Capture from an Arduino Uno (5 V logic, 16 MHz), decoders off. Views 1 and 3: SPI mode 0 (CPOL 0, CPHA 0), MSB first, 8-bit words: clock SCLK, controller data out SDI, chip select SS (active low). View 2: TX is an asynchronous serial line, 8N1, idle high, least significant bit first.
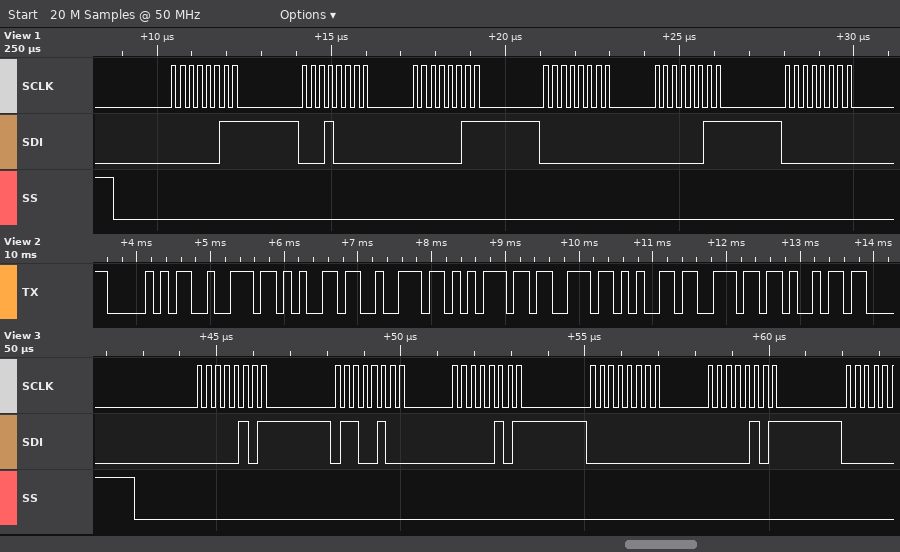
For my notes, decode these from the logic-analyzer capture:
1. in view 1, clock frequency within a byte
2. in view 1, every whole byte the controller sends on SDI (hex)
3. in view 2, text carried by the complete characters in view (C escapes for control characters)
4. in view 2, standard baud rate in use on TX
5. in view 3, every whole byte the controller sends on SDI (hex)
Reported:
4 MHz
03 10 03 00 03 00
"Preruseni"
9600 baud
05 64 05 00 05
